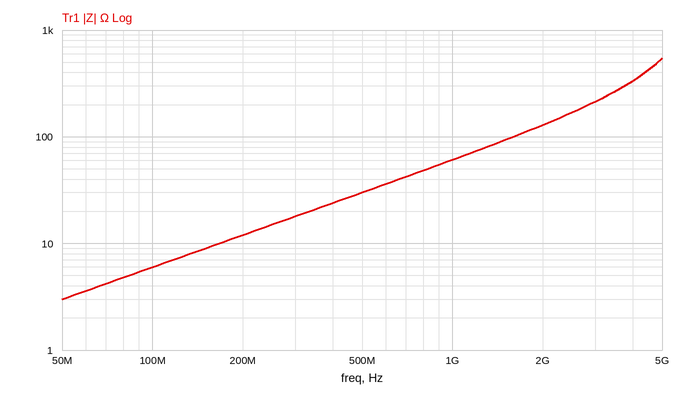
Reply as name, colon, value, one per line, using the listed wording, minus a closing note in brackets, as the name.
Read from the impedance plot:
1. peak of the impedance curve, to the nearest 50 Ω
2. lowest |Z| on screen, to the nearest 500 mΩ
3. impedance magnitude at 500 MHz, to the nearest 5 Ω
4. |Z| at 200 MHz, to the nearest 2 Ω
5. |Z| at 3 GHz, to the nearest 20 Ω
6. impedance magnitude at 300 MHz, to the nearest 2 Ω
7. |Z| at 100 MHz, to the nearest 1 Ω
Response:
peak of the impedance curve, to the nearest 50 Ω: 550 Ω
lowest |Z| on screen, to the nearest 500 mΩ: 3.0 Ω
impedance magnitude at 500 MHz, to the nearest 5 Ω: 30 Ω
|Z| at 200 MHz, to the nearest 2 Ω: 12 Ω
|Z| at 3 GHz, to the nearest 20 Ω: 220 Ω
impedance magnitude at 300 MHz, to the nearest 2 Ω: 18 Ω
|Z| at 100 MHz, to the nearest 1 Ω: 6 Ω
